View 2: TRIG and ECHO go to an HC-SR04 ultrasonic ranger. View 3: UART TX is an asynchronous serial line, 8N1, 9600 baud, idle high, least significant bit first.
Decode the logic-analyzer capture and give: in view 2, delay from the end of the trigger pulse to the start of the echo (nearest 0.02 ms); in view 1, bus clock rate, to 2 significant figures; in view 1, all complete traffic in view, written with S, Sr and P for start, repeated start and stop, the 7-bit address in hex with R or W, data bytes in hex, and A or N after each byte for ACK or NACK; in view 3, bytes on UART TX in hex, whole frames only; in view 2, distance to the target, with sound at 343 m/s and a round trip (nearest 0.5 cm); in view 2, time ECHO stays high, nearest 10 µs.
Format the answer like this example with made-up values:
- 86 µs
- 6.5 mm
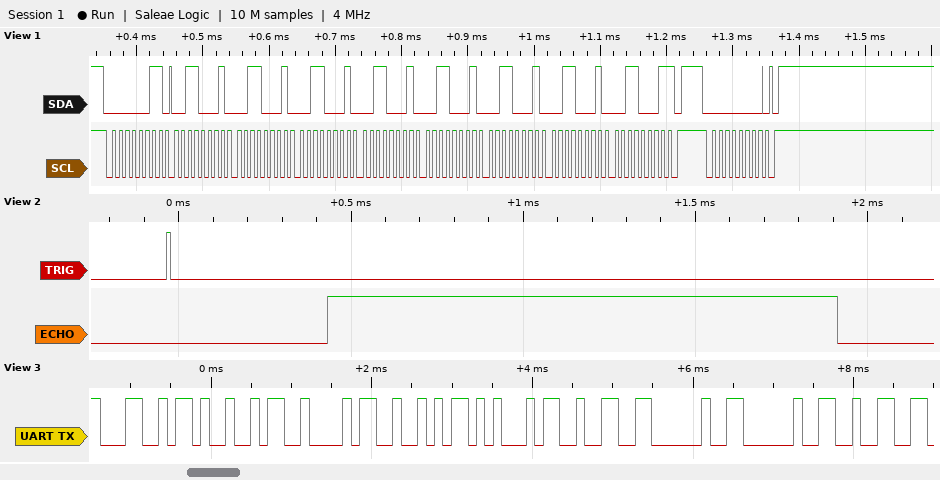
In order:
- 0.46 ms
- 100 kHz
- S 01R A 31 A 31 A 31 A 31 A 31 A 31 A 31 A 31 N P S 00W A P
- 4C 49 42 52 45 32 20 20 32
- 25.5 cm
- 1480 µs
